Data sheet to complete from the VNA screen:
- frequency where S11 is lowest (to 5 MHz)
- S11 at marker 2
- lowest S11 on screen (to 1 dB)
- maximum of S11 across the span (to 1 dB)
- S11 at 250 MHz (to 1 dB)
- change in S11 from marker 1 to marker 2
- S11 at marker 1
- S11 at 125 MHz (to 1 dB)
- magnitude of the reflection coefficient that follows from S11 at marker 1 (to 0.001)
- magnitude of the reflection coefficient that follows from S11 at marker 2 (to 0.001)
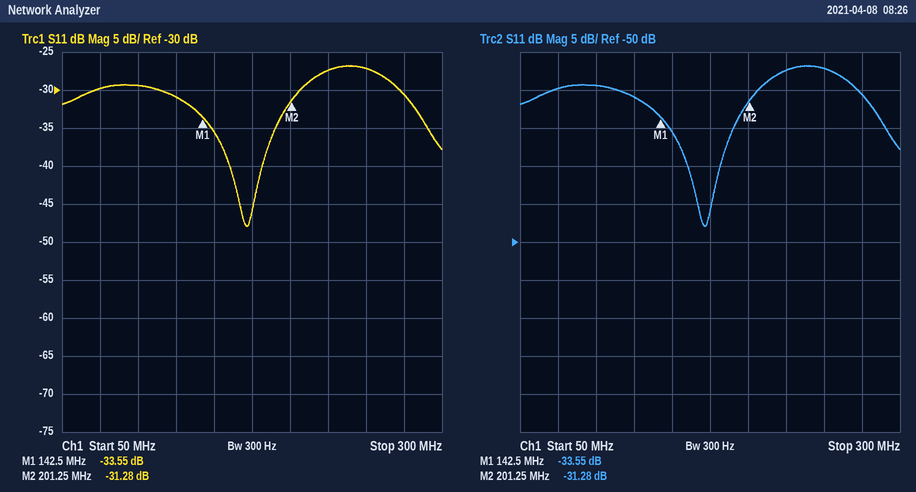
170 MHz
-31.28 dB
-48 dB
-27 dB
-27 dB
2.27 dB
-33.55 dB
-31 dB
0.021
0.027
